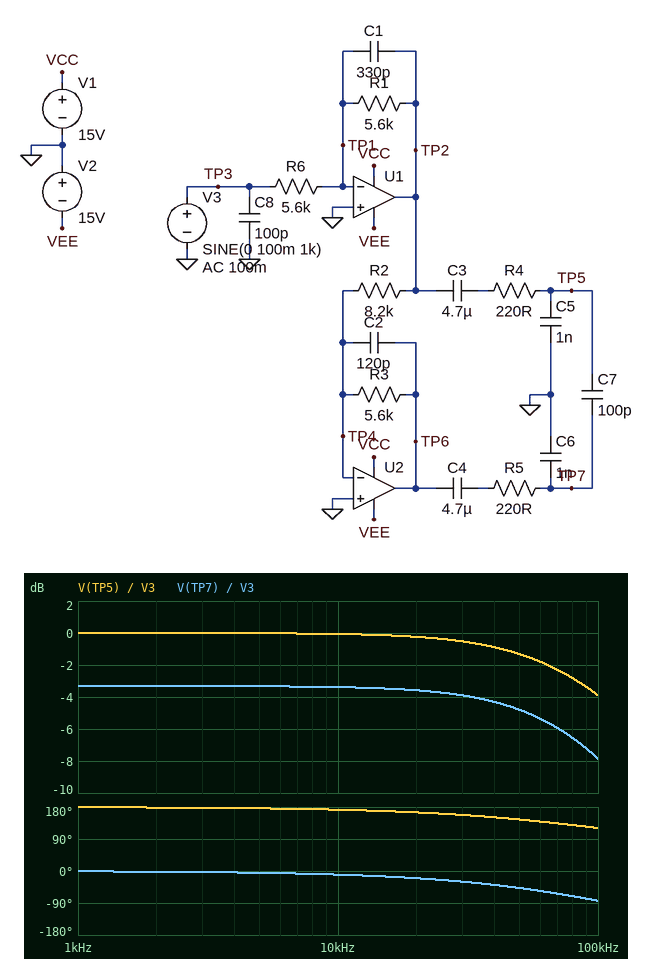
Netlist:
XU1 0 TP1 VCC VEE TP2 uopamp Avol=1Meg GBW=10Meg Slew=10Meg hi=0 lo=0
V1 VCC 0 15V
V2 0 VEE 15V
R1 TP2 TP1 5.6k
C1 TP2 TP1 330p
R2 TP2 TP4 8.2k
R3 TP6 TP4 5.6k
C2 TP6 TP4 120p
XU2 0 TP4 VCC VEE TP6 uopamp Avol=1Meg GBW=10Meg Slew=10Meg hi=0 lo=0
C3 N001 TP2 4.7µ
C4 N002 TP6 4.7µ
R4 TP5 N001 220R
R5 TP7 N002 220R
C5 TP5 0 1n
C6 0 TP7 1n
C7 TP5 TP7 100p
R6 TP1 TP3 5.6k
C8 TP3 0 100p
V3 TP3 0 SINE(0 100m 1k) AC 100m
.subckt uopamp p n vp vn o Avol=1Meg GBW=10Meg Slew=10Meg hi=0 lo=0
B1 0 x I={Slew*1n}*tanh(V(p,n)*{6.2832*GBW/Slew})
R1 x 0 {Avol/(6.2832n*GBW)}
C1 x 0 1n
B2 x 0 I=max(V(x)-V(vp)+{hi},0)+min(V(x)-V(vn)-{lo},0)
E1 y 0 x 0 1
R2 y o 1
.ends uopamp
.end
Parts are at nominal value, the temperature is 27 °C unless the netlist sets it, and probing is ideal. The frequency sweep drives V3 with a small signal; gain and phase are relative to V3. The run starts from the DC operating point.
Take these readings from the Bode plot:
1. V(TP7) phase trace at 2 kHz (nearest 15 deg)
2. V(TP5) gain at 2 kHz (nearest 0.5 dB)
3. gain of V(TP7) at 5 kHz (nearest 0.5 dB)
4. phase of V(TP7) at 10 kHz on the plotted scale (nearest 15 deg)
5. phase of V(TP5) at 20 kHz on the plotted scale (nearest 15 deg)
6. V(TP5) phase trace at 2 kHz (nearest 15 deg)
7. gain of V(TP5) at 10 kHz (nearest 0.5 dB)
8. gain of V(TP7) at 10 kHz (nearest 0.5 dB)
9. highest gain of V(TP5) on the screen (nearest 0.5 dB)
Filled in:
0 deg
0 dB
-3.5 dB
-15 deg
165 deg
180 deg
0 dB
-3.5 dB
0 dB
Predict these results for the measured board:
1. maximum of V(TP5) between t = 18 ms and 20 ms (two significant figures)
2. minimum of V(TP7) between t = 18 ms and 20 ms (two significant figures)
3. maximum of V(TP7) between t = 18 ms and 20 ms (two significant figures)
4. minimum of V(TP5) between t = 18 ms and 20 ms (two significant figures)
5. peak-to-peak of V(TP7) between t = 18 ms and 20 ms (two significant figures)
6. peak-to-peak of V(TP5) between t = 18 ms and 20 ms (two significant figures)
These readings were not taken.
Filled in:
100 mV
-68 mV
68 mV
-100 mV
140 mV
200 mV
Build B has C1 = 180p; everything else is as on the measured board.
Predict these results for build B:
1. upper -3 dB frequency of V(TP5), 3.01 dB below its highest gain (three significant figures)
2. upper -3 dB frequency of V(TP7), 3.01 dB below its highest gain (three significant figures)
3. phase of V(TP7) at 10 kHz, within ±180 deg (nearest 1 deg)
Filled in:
145 kHz
117 kHz
-7 deg
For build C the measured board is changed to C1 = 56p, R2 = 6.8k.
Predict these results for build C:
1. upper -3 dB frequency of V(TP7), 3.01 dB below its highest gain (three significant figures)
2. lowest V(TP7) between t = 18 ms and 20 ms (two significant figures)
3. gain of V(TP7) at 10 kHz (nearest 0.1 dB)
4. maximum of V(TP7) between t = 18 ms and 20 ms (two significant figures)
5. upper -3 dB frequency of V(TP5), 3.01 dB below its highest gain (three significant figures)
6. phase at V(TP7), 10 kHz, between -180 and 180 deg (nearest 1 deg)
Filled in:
188 kHz
-82 mV
-1.7 dB
82 mV
343 kHz
-5 deg
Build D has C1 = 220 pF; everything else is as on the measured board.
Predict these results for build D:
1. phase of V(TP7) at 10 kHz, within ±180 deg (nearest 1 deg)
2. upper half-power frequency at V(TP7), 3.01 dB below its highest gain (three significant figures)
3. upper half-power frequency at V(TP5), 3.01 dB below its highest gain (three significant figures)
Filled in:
-8 deg
103 kHz
122 kHz
